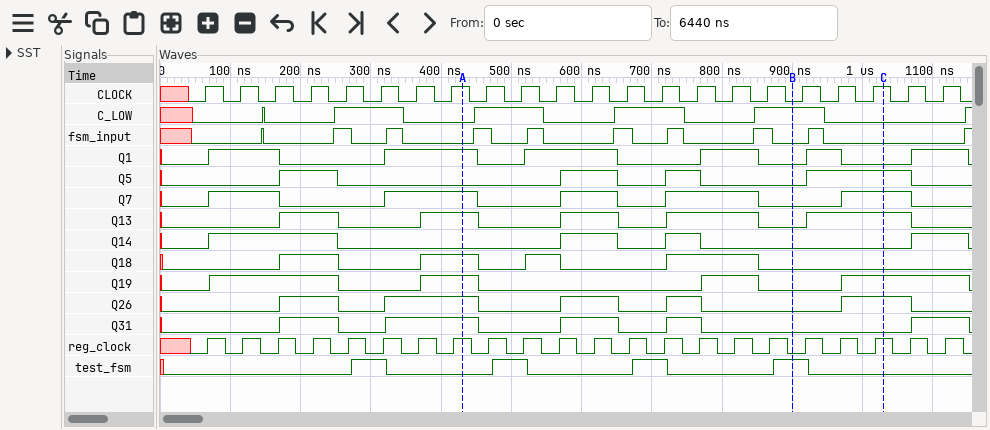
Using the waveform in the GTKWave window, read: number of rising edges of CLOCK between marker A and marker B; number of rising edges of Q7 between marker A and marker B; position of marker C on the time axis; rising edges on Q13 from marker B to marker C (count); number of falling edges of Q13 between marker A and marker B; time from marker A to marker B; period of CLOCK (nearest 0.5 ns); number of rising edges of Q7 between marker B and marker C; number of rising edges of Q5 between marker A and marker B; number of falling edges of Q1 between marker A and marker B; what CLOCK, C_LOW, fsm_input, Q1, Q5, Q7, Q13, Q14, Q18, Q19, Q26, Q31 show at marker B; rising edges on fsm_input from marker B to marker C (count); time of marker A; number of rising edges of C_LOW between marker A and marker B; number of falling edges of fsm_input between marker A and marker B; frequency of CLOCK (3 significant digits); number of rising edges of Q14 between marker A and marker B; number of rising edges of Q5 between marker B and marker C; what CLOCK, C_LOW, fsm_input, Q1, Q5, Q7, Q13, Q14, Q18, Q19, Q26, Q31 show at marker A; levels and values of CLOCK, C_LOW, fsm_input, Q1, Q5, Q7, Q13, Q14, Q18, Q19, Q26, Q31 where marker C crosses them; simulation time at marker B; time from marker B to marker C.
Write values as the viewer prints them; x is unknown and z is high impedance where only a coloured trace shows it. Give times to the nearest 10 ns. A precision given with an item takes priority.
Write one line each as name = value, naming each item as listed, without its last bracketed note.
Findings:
number of rising edges of CLOCK between marker A and marker B = 9
number of rising edges of Q7 between marker A and marker B = 2
position of marker C on the time axis = 1030 ns
rising edges on Q13 from marker B to marker C = 1
number of falling edges of Q13 between marker A and marker B = 3
time from marker A to marker B = 470 ns
period of CLOCK = 50 ns
number of rising edges of Q7 between marker B and marker C = 1
number of rising edges of Q5 between marker A and marker B = 2
number of falling edges of Q1 between marker A and marker B = 3
what CLOCK, C_LOW, fsm_input, Q1, Q5, Q7, Q13, Q14, Q18, Q19, Q26, Q31 show at marker B = CLOCK=0, C_LOW=1, fsm_input=0, Q1=0, Q5=0, Q7=0, Q13=0, Q14=0, Q18=0, Q19=0, Q26=0, Q31=0
rising edges on fsm_input from marker B to marker C = 1
time of marker A = 430 ns
number of rising edges of C_LOW between marker A and marker B = 3
number of falling edges of fsm_input between marker A and marker B = 5
frequency of CLOCK = 20.0 MHz
number of rising edges of Q14 between marker A and marker B = 2
number of rising edges of Q5 between marker B and marker C = 1
what CLOCK, C_LOW, fsm_input, Q1, Q5, Q7, Q13, Q14, Q18, Q19, Q26, Q31 show at marker A = CLOCK=1, C_LOW=0, fsm_input=0, Q1=1, Q5=0, Q7=1, Q13=1, Q14=0, Q18=1, Q19=1, Q26=1, Q31=1
levels and values of CLOCK, C_LOW, fsm_input, Q1, Q5, Q7, Q13, Q14, Q18, Q19, Q26, Q31 where marker C crosses them = CLOCK=1, C_LOW=0, fsm_input=0, Q1=0, Q5=1, Q7=1, Q13=1, Q14=0, Q18=0, Q19=1, Q26=1, Q31=0
simulation time at marker B = 900 ns
time from marker B to marker C = 130 ns
